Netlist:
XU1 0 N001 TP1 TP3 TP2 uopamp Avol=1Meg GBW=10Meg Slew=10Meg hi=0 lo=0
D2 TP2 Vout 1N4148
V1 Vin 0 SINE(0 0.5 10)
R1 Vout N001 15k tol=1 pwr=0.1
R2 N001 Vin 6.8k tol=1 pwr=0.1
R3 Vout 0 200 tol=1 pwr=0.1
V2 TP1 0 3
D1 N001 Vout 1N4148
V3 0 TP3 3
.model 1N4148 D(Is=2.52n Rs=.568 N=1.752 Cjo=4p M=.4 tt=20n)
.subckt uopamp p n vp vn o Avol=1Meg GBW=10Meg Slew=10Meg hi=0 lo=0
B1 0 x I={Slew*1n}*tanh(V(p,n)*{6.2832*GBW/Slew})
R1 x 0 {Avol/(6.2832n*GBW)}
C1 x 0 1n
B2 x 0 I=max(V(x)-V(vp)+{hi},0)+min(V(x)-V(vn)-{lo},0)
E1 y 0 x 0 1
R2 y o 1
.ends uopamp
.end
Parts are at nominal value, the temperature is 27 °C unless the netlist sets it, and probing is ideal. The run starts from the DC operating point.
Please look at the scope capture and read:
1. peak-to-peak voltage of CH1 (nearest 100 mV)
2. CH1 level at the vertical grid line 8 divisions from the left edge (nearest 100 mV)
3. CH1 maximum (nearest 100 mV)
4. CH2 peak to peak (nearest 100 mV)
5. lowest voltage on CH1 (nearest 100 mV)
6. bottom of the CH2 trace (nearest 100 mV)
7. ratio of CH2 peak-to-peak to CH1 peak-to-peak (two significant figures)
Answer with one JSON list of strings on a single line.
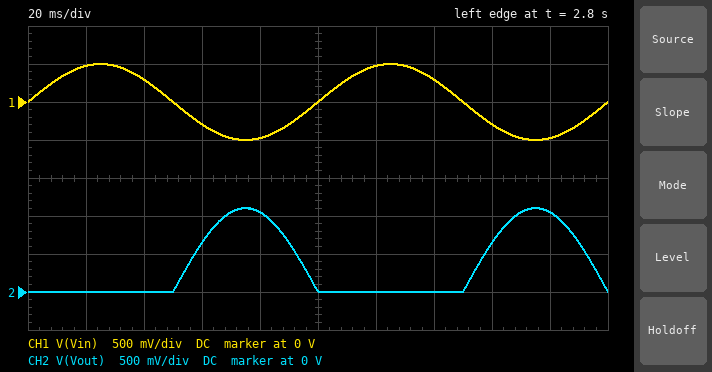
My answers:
["1.0 V", "-300 mV", "500 mV", "1.1 V", "-500 mV", "0 V", "1.1"]
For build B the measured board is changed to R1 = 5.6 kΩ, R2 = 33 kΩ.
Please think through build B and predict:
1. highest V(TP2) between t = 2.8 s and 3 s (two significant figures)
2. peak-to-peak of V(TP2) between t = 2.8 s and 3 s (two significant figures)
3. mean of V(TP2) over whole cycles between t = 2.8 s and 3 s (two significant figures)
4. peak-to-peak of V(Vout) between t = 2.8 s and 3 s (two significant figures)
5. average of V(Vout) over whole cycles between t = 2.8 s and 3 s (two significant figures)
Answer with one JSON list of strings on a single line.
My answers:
["630 mV", "3.6 V", "-1.2 V", "85 mV", "28 mV"]
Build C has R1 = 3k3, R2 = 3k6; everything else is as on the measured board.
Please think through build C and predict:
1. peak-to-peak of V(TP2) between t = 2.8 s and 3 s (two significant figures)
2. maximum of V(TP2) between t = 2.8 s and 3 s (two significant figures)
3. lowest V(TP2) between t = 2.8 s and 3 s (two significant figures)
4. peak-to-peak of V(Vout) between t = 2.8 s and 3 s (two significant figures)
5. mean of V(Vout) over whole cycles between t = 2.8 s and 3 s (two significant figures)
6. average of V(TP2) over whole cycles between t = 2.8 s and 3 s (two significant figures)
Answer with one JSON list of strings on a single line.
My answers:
["4.1 V", "1.1 V", "-3.0 V", "460 mV", "150 mV", "-1.1 V"]
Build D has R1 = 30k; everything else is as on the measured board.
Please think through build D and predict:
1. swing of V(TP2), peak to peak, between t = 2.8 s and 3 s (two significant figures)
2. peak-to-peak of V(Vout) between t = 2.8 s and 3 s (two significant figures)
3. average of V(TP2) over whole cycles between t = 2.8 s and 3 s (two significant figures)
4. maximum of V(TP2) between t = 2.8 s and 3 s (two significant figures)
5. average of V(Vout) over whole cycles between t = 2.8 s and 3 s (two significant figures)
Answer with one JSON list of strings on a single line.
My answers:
["5.9 V", "2.2 V", "-470 mV", "2.9 V", "700 mV"]
